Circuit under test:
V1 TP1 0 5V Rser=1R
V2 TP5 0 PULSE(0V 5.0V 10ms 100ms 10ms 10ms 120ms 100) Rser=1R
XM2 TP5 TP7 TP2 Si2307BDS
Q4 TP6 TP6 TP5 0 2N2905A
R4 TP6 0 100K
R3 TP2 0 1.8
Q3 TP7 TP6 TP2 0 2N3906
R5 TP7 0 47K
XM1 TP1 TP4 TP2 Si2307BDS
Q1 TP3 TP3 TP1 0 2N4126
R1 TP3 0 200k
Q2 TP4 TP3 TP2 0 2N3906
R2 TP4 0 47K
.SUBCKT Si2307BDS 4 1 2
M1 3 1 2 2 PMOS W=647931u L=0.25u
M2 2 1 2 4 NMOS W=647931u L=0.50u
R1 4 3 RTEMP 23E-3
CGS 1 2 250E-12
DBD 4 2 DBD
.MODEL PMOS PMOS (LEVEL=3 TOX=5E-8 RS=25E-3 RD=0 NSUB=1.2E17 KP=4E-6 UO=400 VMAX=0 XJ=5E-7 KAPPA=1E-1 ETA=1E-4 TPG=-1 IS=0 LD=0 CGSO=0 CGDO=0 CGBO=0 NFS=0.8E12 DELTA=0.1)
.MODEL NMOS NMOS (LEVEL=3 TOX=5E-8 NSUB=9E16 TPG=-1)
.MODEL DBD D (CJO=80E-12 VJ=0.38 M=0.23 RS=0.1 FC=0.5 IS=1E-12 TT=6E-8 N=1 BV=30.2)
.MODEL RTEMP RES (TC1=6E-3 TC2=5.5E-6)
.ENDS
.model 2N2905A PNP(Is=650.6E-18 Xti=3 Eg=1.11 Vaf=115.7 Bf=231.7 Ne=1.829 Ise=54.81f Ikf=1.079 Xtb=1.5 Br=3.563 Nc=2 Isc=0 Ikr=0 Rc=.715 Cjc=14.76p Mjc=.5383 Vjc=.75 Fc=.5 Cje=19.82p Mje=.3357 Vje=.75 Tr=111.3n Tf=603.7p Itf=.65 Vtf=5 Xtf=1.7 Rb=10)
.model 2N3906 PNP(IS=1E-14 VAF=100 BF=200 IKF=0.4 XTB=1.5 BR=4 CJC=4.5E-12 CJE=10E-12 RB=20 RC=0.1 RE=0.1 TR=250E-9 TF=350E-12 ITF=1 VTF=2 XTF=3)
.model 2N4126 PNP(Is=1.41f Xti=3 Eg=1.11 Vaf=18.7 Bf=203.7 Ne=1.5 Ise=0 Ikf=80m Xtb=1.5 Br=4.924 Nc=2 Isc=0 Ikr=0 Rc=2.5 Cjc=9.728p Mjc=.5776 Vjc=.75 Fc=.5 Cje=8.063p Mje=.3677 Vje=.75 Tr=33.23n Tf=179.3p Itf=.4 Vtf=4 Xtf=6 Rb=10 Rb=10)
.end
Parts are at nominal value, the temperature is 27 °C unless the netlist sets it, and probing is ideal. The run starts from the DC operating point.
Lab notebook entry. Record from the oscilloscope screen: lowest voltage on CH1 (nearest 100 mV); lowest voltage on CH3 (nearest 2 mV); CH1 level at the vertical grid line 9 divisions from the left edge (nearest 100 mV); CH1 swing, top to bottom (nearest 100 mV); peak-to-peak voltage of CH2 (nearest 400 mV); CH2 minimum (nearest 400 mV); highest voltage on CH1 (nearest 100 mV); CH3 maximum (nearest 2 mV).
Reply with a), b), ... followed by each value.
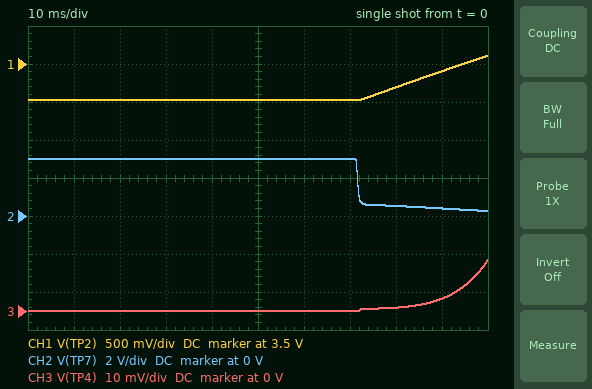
a) 3.0 V
b) 0 V
c) 3.4 V
d) 600 mV
e) 2.8 V
f) 400 mV
g) 3.6 V
h) 14 mV
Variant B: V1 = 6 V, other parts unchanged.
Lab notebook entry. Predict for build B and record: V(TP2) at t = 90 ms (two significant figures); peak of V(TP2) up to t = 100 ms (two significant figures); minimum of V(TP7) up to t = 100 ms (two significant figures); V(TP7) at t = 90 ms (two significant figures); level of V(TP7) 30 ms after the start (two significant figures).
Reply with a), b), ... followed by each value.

a) 3.8 V
b) 4.0 V
c) 960 mV
d) 1.2 V
e) 3.7 V
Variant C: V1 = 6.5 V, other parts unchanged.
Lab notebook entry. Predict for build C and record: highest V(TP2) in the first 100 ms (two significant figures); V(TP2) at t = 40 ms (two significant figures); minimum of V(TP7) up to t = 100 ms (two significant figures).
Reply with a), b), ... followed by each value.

a) 4.2 V
b) 4.0 V
c) 1.4 V
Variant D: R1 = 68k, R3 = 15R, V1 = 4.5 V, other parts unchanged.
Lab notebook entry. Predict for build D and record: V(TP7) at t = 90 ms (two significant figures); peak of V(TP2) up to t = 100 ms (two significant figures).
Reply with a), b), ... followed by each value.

a) 4.1 V
b) 4.3 V
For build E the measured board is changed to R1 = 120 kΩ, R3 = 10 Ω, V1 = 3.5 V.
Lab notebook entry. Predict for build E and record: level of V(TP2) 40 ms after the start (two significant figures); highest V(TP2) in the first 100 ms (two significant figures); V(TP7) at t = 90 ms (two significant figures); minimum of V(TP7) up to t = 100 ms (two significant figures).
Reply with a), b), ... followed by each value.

a) 3.1 V
b) 4.0 V
c) 670 mV
d) 600 mV
